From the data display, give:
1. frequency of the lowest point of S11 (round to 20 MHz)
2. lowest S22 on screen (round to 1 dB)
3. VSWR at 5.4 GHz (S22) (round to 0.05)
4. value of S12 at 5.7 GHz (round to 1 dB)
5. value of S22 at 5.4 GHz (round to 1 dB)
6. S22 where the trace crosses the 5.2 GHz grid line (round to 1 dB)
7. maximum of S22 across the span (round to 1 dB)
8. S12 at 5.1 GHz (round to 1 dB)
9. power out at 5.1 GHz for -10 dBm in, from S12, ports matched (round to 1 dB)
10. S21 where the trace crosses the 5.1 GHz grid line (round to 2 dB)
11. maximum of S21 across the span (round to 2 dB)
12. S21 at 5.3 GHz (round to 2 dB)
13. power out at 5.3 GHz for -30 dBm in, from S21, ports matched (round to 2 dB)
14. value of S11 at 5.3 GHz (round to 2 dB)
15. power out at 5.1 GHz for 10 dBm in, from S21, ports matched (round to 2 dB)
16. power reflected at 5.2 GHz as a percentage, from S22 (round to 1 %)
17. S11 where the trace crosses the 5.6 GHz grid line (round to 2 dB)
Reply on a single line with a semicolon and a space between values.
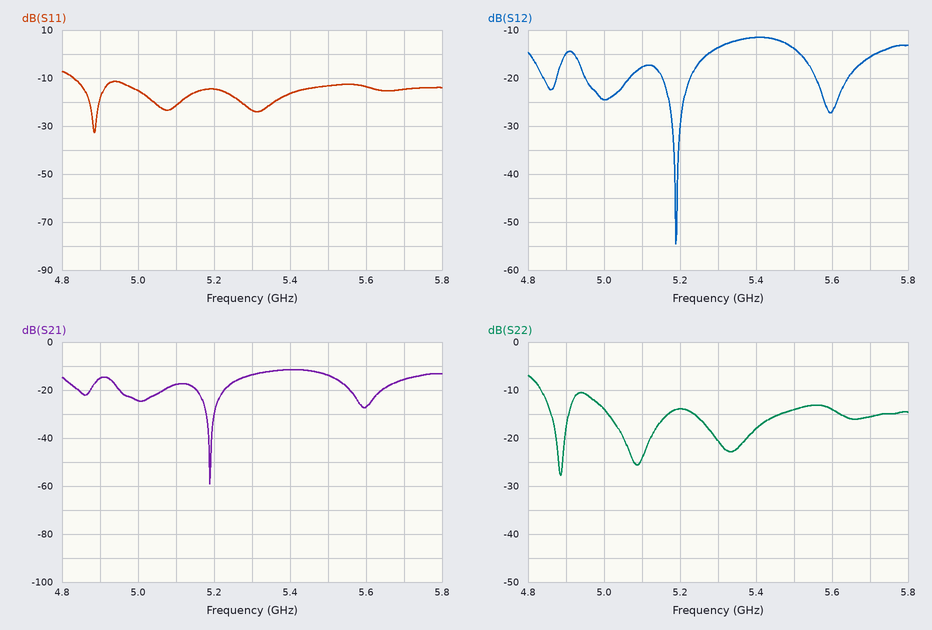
4.88 GHz; -28 dB; 1.30; -16 dB; -18 dB; -14 dB; -7 dB; -18 dB; -28 dBm; -18 dB; -12 dB; -14 dB; -44 dBm; -24 dB; -8 dBm; 4 %; -14 dB
